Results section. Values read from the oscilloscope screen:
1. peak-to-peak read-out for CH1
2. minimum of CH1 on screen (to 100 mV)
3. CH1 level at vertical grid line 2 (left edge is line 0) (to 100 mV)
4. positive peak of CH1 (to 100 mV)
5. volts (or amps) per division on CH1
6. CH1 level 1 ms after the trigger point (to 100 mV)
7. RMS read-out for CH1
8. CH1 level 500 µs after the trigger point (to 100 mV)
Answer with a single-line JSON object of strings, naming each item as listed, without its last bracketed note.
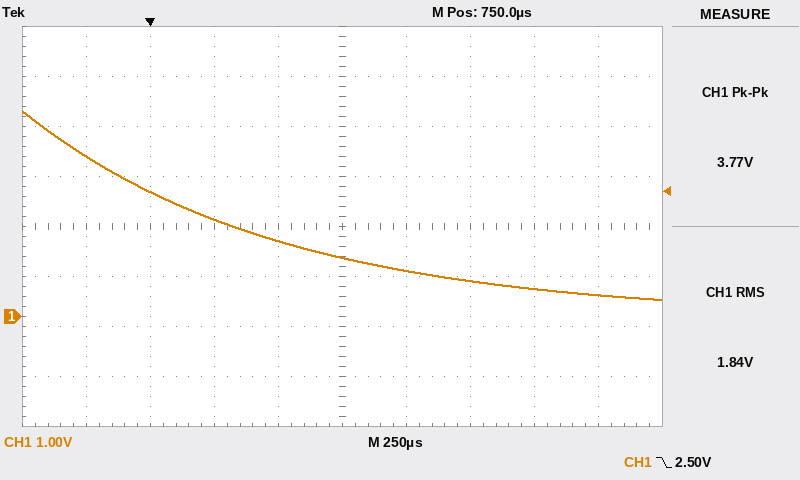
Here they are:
{"peak-to-peak read-out for CH1": "3.77 V", "minimum of CH1 on screen": "300 mV", "CH1 level at vertical grid line 2 (left edge is line 0)": "2.5 V", "positive peak of CH1": "4.1 V", "volts (or amps) per division on CH1": "1 V", "CH1 level 1 ms after the trigger point": "900 mV", "RMS read-out for CH1": "1.84 V", "CH1 level 500 µs after the trigger point": "1.5 V"}
